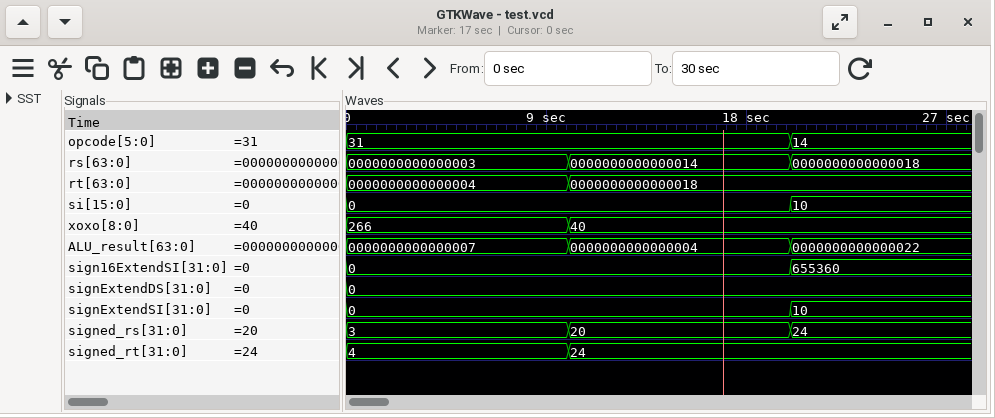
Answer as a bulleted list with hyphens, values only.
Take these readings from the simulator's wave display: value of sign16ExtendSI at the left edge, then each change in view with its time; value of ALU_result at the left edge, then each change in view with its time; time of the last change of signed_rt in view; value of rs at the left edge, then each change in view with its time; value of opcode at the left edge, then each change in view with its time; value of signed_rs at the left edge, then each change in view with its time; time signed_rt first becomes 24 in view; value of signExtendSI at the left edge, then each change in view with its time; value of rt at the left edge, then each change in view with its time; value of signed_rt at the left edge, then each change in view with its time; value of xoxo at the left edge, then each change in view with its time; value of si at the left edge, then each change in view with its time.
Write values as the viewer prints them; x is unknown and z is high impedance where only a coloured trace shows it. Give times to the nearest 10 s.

- 0, 655360 at 20 s
- 0000000000000007, 0000000000000004 at 10 s, 0000000000000022 at 20 s
- 10 s
- 0000000000000003, 0000000000000014 at 10 s, 0000000000000018 at 20 s
- 31, 14 at 20 s
- 3, 20 at 10 s, 24 at 20 s
- 10 s
- 0, 10 at 20 s
- 0000000000000004, 0000000000000018 at 10 s
- 4, 24 at 10 s
- 266, 40 at 10 s
- 0, 10 at 20 s
